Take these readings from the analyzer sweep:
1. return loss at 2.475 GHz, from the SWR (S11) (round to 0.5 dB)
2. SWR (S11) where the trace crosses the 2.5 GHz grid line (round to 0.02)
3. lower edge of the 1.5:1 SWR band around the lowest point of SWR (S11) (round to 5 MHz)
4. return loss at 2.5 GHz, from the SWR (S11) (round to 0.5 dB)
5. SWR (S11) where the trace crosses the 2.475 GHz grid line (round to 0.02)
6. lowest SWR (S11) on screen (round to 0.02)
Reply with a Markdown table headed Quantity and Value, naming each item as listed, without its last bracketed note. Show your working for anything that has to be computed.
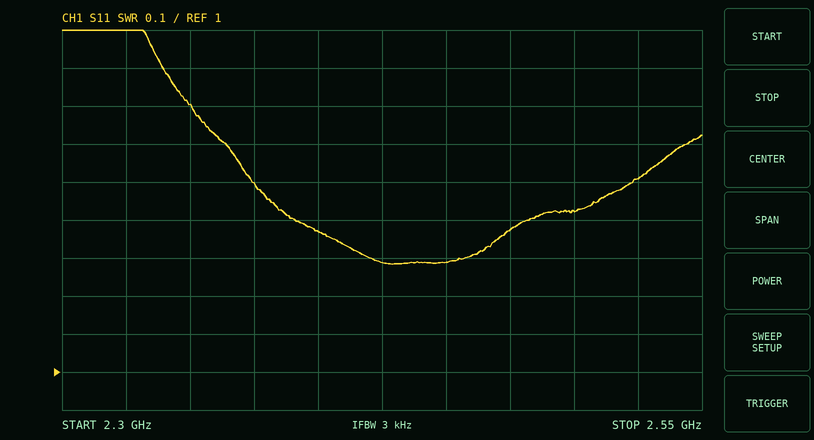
| Quantity | Value |
|---|---|
| return loss at 2.475 GHz, from the SWR (S11) | −20 log10((1.38 − 1)/(1.38 + 1)) ≈ 15.9 dB, so 16.0 dB to the nearest 0.5 dB |
| SWR (S11) where the trace crosses the 2.5 GHz grid line | 1.42 |
| lower edge of the 1.5:1 SWR band around the lowest point of SWR (S11) | 2.375 GHz |
| return loss at 2.5 GHz, from the SWR (S11) | −20 log10((1.42 − 1)/(1.42 + 1)) ≈ 15.2 dB, so 15.0 dB to the nearest 0.5 dB |
| SWR (S11) where the trace crosses the 2.475 GHz grid line | 1.38 |
| lowest SWR (S11) on screen | 1.28 |
